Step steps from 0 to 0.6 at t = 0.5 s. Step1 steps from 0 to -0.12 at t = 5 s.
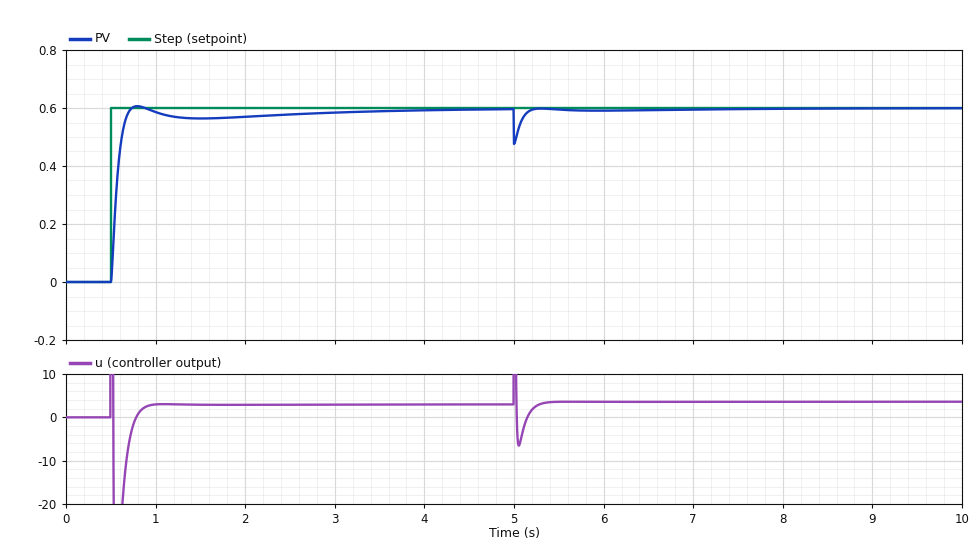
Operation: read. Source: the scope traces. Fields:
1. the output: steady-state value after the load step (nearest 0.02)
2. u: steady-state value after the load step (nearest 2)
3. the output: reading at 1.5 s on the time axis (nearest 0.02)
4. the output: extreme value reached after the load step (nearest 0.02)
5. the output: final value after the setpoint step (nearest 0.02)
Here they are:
0.60
4
0.56
0.48
0.60
